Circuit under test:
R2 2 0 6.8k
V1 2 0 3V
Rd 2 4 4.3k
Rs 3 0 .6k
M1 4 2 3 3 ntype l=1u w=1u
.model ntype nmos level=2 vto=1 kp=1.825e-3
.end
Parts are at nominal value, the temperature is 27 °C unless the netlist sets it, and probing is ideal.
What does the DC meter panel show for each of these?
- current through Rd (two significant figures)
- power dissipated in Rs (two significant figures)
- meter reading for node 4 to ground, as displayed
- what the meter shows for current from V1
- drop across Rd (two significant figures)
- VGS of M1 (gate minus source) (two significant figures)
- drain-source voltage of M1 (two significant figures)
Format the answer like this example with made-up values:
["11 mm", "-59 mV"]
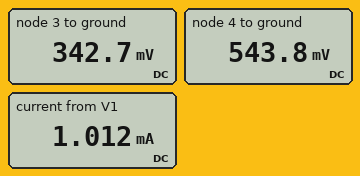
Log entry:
["570 µA", "200 µW", "543.8 mV", "1.012 mA", "2.5 V", "2.7 V", "200 mV"]
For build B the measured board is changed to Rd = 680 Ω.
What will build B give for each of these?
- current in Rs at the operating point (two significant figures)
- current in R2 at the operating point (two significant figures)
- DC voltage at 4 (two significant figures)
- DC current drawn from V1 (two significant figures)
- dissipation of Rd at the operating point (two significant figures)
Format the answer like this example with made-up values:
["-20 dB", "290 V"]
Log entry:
["1.3 mA", "440 µA", "2.1 V", "1.8 mA", "1.2 mW"]
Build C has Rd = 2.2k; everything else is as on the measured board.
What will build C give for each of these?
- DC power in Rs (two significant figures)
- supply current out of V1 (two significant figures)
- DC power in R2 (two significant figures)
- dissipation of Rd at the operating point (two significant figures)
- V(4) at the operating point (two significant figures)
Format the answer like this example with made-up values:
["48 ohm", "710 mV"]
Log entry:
["510 µW", "1.4 mA", "1.3 mW", "1.9 mW", "960 mV"]
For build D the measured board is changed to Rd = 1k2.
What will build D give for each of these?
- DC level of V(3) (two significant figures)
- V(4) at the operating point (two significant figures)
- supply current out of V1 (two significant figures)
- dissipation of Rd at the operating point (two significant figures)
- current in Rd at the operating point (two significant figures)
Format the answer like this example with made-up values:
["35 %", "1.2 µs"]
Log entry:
["740 mV", "1.5 V", "1.7 mA", "1.8 mW", "1.2 mA"]
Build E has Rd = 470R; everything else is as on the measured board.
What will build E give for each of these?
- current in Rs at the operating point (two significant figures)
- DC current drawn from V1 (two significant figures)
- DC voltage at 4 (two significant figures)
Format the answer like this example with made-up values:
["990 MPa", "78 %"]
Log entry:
["1.3 mA", "1.8 mA", "2.4 V"]
